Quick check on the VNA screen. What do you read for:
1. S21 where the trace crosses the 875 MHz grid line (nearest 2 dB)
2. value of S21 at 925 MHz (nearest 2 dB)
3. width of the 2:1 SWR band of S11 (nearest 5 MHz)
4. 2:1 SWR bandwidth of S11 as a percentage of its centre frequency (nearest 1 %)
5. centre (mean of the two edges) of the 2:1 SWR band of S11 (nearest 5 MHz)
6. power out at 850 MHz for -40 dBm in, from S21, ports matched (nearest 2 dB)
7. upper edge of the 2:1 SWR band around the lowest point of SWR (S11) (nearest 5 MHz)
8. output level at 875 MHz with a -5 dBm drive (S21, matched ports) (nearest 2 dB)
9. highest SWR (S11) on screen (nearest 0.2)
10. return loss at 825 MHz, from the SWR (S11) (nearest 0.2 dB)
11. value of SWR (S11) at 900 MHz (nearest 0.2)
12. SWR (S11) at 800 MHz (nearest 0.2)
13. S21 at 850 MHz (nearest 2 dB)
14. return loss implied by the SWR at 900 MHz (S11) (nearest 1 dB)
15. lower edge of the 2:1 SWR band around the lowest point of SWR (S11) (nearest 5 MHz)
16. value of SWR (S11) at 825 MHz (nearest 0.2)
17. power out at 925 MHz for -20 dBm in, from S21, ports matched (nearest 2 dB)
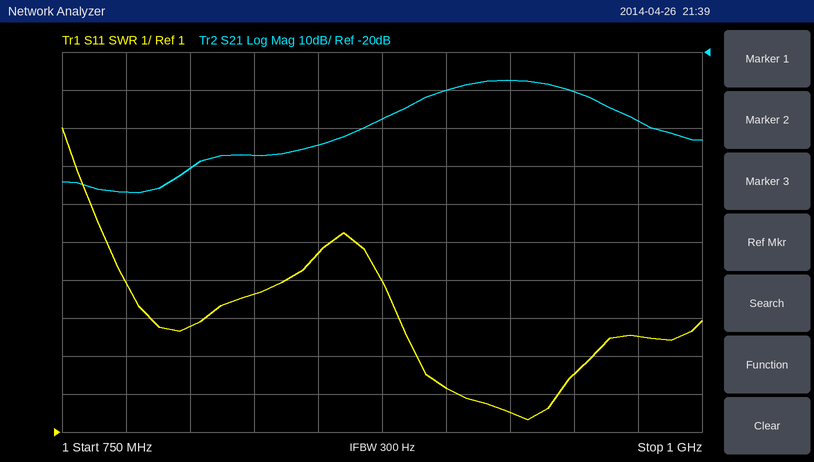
-38 dB
-28 dB
40 MHz
4 %
925 MHz
-84 dBm
945 MHz
-42 dBm
9.0
3.8 dB
2.2
3.8
-44 dB
9 dB
905 MHz
4.6
-48 dBm
